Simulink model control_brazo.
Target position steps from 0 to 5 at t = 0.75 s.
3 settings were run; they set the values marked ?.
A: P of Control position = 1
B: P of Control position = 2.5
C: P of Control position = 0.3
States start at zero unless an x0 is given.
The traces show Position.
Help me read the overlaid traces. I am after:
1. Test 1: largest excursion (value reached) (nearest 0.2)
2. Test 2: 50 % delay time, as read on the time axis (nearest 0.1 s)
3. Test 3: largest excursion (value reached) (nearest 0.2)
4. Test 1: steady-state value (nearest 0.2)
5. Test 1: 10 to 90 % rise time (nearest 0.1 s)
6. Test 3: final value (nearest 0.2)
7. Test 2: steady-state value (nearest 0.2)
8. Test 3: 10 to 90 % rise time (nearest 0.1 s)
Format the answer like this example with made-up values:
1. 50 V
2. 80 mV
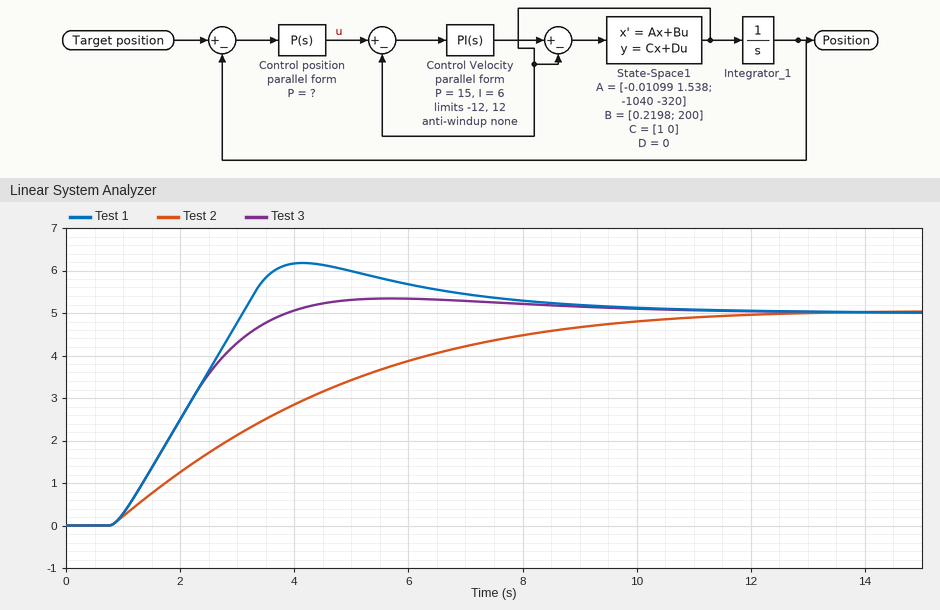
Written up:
1. 6.2
2. 3.5 s
3. 5.4
4. 5.0
5. 1.8 s
6. 5.0
7. 5.0
8. 2.1 s
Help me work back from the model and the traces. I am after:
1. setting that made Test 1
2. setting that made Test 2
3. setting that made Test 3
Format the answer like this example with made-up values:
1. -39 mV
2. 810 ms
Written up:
1. B
2. C
3. A
